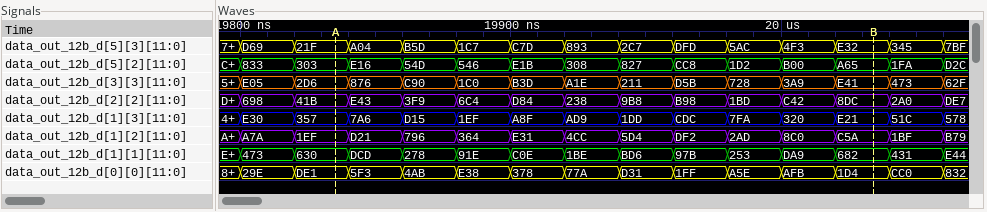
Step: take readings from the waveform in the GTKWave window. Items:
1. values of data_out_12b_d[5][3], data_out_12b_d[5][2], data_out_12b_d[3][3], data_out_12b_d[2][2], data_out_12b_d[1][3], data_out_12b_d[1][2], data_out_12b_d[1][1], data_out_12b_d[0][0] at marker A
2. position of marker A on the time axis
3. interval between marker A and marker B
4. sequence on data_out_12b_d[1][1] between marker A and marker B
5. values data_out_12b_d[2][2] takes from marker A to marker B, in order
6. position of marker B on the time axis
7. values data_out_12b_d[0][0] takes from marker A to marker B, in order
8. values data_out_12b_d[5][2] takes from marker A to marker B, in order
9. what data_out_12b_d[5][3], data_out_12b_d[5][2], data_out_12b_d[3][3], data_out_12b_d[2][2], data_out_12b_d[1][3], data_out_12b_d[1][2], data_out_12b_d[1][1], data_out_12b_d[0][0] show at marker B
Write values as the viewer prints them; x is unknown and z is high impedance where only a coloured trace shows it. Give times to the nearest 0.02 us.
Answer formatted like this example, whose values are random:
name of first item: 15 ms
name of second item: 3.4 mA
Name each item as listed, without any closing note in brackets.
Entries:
values of data_out_12b_d[5][3], data_out_12b_d[5][2], data_out_12b_d[3][3], data_out_12b_d[2][2], data_out_12b_d[1][3], data_out_12b_d[1][2], data_out_12b_d[1][1], data_out_12b_d[0][0] at marker A: data_out_12b_d[5][3]=21F, data_out_12b_d[5][2]=303, data_out_12b_d[3][3]=2D6, data_out_12b_d[2][2]=41B, data_out_12b_d[1][3]=357, data_out_12b_d[1][2]=1EF, data_out_12b_d[1][1]=630, data_out_12b_d[0][0]=DE1
position of marker A on the time axis: 19.84 us
interval between marker A and marker B: 0.2 us
sequence on data_out_12b_d[1][1] between marker A and marker B: 630, DCD, 278, 91E, C0E, 1BE, BD6, 97B, 253, DA9, 682
values data_out_12b_d[2][2] takes from marker A to marker B, in order: 41B, E43, 3F9, 6C4, D84, 238, 9B8, B98, 1BD, C42, 8DC
position of marker B on the time axis: 20.04 us
values data_out_12b_d[0][0] takes from marker A to marker B, in order: DE1, 5F3, 4AB, E38, 378, 77A, D31, 1FF, A5E, AFB, 1D4
values data_out_12b_d[5][2] takes from marker A to marker B, in order: 303, E16, 54D, 546, E1B, 308, 827, CC8, 1D2, B00, A65
what data_out_12b_d[5][3], data_out_12b_d[5][2], data_out_12b_d[3][3], data_out_12b_d[2][2], data_out_12b_d[1][3], data_out_12b_d[1][2], data_out_12b_d[1][1], data_out_12b_d[0][0] show at marker B: data_out_12b_d[5][3]=E32, data_out_12b_d[5][2]=A65, data_out_12b_d[3][3]=E41, data_out_12b_d[2][2]=8DC, data_out_12b_d[1][3]=E21, data_out_12b_d[1][2]=C5A, data_out_12b_d[1][1]=682, data_out_12b_d[0][0]=1D4
